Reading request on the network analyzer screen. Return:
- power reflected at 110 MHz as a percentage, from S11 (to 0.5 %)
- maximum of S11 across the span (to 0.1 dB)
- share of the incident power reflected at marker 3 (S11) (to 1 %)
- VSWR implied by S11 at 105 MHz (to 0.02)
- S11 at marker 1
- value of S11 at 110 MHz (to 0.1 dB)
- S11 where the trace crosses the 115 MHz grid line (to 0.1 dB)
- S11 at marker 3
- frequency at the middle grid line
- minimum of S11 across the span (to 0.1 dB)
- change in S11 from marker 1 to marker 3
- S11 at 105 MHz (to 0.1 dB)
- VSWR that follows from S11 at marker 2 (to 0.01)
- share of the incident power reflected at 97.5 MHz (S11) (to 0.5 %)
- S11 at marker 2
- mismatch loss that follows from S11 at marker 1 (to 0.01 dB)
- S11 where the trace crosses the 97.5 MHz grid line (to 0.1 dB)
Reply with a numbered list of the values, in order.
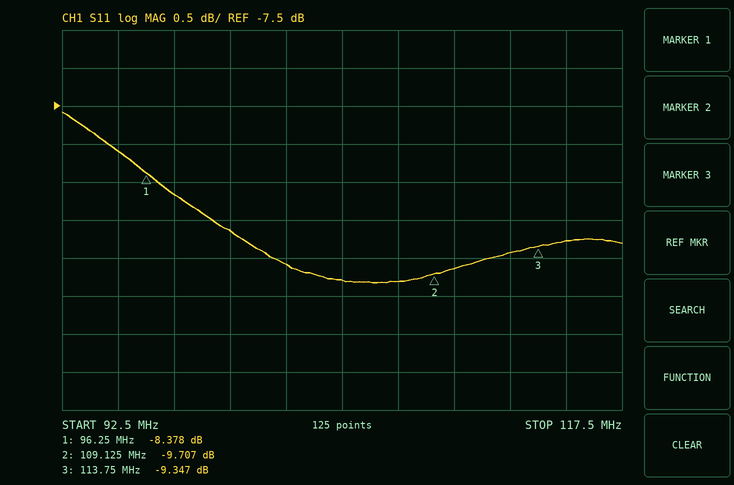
1. 11.0 %
2. -7.6 dB
3. 12 %
4. 1.96
5. -8.378 dB
6. -9.6 dB
7. -9.3 dB
8. -9.347 dB
9. 105 MHz
10. -9.8 dB
11. -0.969 dB
12. -9.8 dB
13. 1.97
14. 13.5 %
15. -9.707 dB
16. 0.68 dB
17. -8.7 dB
